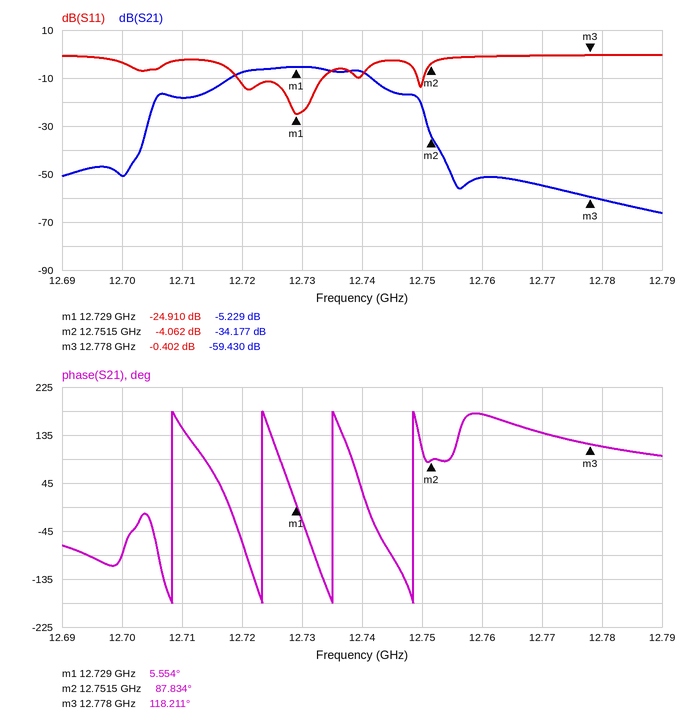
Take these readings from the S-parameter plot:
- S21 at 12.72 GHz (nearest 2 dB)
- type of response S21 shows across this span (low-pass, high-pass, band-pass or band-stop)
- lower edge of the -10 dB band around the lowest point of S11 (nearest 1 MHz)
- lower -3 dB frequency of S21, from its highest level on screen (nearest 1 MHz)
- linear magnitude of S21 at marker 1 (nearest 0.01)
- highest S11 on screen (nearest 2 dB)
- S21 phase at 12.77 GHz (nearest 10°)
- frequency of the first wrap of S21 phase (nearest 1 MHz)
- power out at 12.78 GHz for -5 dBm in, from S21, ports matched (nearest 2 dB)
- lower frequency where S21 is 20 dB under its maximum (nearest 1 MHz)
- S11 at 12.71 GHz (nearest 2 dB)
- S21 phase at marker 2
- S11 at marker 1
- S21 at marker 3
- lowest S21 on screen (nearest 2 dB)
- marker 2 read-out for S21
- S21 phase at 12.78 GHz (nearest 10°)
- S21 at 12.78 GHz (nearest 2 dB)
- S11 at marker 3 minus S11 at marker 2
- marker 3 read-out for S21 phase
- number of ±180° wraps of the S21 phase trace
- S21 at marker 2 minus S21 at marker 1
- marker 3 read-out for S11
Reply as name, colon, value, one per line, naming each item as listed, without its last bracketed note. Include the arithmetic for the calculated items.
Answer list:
S21 at 12.72 GHz: -8 dB
type of response S21 shows across this span: band-pass
lower edge of the -10 dB band around the lowest point of S11: 12.719 GHz
lower -3 dB frequency of S21, from its highest level on screen: 12.719 GHz
linear magnitude of S21 at marker 1: 10^(-5.229/20) ≈ 0.55
highest S11 on screen: 0 dB
S21 phase at 12.77 GHz: 140°
frequency of the first wrap of S21 phase: 12.708 GHz
power out at 12.78 GHz for -5 dBm in, from S21, ports matched: -5 dBm + (-60 dB) = -66 dBm
lower frequency where S21 is 20 dB under its maximum: 12.705 GHz
S11 at 12.71 GHz: -2 dB
S21 phase at marker 2: 87.834°
S11 at marker 1: -24.910 dB
S21 at marker 3: -59.430 dB
lowest S21 on screen: -66 dB
marker 2 read-out for S21: -34.177 dB
S21 phase at 12.78 GHz: 110°
S21 at 12.78 GHz: -60 dB
S11 at marker 3 minus S11 at marker 2: -0.402 − (-4.062) = 3.660 dB
marker 3 read-out for S21 phase: 118.211°
number of ±180° wraps of the S21 phase trace: 4
S21 at marker 2 minus S21 at marker 1: -34.177 − (-5.229) = -28.948 dB
marker 3 read-out for S11: -0.402 dB
